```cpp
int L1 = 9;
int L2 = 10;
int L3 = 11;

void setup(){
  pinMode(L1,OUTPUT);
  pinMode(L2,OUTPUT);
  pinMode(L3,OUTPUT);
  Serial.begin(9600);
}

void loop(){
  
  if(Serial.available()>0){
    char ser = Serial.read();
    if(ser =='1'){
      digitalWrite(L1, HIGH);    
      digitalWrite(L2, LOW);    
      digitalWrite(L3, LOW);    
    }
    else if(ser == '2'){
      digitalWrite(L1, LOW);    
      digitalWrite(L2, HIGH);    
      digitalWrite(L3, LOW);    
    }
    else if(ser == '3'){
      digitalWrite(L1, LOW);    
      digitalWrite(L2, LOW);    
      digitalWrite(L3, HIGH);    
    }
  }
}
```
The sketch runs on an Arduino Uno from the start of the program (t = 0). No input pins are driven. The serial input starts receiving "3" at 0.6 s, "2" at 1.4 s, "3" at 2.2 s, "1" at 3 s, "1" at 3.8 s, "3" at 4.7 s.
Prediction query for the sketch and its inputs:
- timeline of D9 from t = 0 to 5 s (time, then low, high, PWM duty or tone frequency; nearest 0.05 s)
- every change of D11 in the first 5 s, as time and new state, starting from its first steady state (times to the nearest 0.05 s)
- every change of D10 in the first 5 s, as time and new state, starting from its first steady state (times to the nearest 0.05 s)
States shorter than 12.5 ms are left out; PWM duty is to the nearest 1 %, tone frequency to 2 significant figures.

0 s low; 3 s high; 4.7 s low
0 s low; 0.6 s high; 1.4 s low; 2.2 s high; 3 s low; 4.7 s high
0 s low; 1.4 s high; 2.2 s low
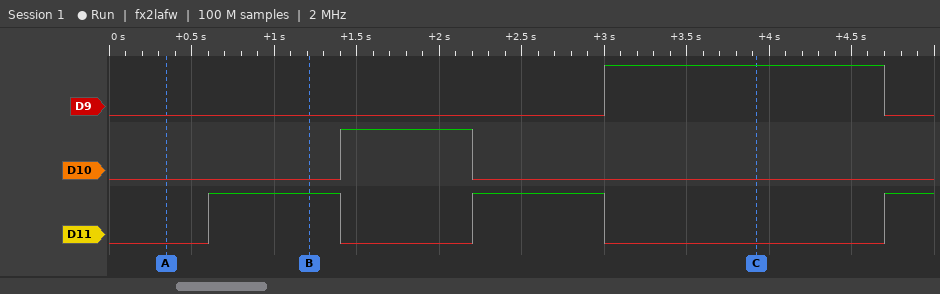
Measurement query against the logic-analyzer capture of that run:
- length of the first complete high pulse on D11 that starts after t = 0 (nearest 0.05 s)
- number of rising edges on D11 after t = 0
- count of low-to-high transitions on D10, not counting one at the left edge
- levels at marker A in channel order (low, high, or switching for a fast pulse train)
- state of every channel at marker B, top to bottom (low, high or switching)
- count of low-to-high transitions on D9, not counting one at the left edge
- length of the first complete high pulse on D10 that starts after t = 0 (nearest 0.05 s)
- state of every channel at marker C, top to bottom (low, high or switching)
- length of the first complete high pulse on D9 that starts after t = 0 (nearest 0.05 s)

0.80 s
3
1
D9 low, D10 low, D11 low
D9 low, D10 low, D11 high
1
0.80 s
D9 high, D10 low, D11 low
1.70 s
